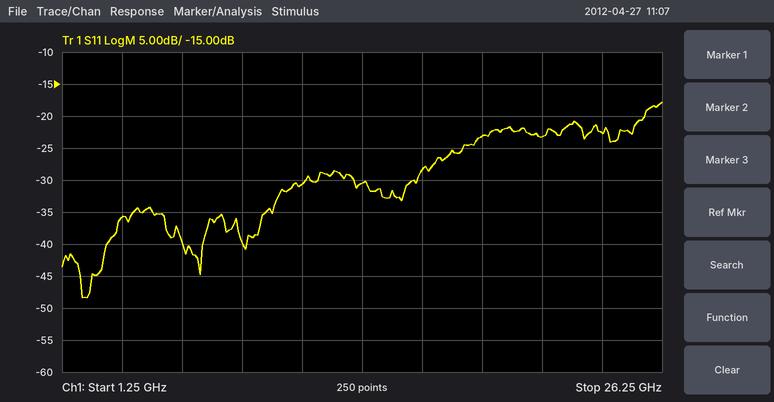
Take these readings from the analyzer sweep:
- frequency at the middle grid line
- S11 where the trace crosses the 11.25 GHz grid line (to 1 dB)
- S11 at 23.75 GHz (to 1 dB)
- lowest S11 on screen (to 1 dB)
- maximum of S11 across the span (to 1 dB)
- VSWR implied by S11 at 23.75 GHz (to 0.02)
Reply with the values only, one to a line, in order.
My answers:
13.75 GHz
-31 dB
-23 dB
-48 dB
-18 dB
1.16
